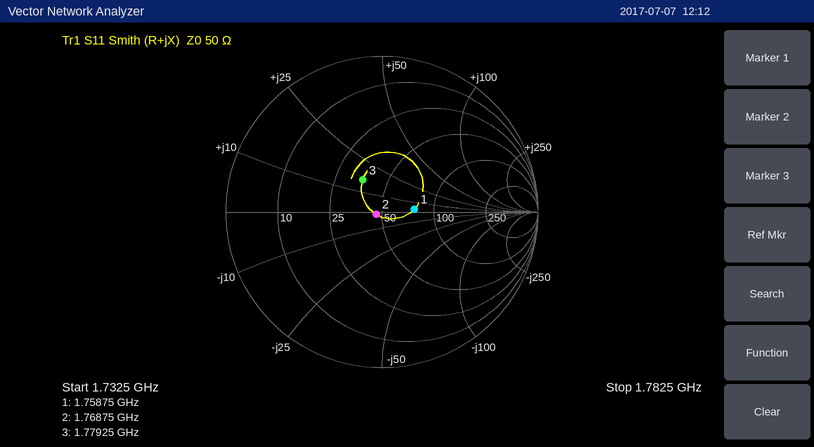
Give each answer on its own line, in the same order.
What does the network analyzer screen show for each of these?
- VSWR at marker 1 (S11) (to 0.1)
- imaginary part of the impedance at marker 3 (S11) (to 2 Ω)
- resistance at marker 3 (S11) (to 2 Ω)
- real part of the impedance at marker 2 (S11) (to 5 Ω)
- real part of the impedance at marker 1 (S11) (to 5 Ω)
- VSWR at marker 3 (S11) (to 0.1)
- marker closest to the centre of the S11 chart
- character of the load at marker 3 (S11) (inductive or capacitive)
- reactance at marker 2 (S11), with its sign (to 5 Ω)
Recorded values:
1.5
+16 Ω
36 Ω
45 Ω
75 Ω
1.6
marker 2
inductive
0 Ω
